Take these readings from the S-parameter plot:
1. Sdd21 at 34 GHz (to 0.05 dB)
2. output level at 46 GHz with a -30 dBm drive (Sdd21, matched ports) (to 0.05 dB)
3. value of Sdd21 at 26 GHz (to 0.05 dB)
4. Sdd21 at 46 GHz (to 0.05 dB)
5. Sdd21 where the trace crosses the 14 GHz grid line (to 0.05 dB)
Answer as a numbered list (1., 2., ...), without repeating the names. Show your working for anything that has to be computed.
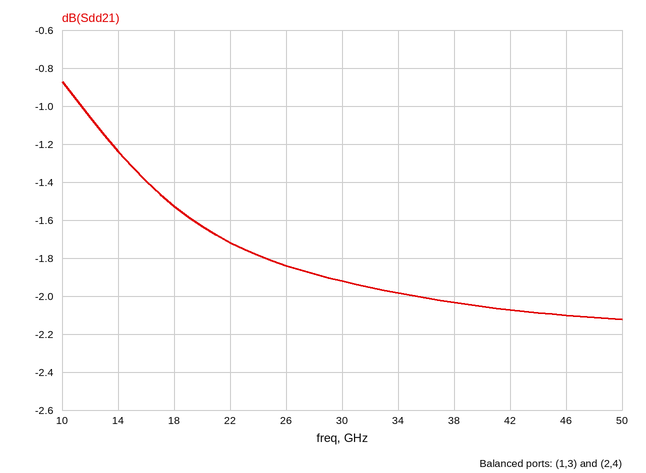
1. -2.00 dB
2. -30 dBm + (-2.10 dB) = -32.10 dBm
3. -1.85 dB
4. -2.10 dB
5. -1.25 dB
